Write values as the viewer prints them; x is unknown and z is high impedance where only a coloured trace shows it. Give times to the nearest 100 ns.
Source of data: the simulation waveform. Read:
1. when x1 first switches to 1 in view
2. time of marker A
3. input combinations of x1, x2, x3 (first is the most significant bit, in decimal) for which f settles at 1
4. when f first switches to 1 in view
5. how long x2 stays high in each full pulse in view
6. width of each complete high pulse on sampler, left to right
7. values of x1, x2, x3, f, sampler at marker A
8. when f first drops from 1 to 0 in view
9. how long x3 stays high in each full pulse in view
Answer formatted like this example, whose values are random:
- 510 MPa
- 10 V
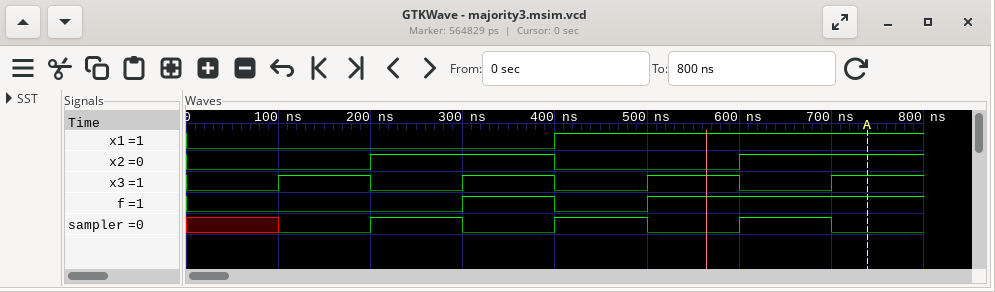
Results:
- 400 ns
- 700 ns
- 3, 5, 6, 7
- 300 ns
- 200 ns
- 100 ns, 100 ns, 100 ns
- x1=1, x2=1, x3=1, f=1, sampler=0
- 400 ns
- 100 ns, 100 ns, 100 ns
